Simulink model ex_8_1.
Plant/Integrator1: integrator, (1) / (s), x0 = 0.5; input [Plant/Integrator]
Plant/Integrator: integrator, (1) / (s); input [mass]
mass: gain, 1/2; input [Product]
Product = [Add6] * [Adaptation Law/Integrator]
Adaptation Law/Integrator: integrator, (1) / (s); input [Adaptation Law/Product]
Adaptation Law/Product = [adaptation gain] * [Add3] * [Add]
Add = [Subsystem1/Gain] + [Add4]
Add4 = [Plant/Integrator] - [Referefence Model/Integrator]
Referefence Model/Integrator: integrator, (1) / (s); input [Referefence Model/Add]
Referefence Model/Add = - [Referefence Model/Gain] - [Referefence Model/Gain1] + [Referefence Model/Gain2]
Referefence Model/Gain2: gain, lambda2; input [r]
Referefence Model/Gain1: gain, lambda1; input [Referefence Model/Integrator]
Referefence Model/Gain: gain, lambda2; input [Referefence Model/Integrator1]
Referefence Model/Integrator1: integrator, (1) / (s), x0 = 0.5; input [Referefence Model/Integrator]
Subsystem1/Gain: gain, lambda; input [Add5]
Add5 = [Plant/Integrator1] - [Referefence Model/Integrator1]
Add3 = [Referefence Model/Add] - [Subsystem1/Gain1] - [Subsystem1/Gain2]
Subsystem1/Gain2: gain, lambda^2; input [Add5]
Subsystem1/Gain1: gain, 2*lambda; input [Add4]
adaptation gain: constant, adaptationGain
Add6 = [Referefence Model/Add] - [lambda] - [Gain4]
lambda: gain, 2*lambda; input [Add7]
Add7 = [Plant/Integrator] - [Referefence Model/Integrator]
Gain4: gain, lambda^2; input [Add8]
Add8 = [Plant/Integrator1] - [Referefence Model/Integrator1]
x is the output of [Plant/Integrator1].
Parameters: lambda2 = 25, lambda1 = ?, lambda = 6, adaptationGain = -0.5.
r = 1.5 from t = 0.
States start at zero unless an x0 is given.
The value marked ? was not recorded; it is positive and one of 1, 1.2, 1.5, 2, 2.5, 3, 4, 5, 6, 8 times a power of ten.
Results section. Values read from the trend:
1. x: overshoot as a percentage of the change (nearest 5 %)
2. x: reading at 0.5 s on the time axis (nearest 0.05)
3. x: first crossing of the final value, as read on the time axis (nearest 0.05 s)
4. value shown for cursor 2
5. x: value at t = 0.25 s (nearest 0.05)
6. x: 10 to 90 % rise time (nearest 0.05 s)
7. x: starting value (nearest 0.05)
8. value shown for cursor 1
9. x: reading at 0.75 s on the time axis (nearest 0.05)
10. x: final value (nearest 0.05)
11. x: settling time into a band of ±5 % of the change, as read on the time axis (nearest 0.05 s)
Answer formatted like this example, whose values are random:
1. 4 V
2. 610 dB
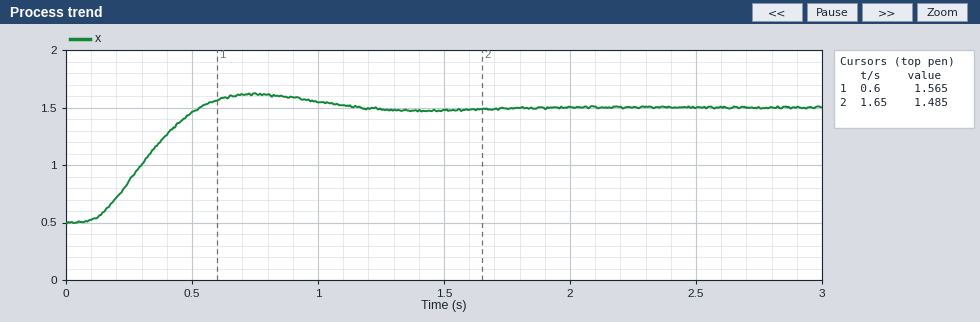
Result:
1. 10 %
2. 1.45
3. 0.55 s
4. 1.485
5. 0.85
6. 0.30 s
7. 0.50
8. 1.565
9. 1.60
10. 1.50
11. 1.00 s
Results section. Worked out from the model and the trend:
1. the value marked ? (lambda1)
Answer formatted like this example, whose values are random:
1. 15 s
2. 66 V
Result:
1. 5
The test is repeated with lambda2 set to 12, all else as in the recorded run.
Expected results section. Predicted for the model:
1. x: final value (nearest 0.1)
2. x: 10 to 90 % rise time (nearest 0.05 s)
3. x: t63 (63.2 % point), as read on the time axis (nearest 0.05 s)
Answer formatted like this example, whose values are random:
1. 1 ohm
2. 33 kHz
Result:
1. 1.5
2. 0.55 s
3. 0.55 s
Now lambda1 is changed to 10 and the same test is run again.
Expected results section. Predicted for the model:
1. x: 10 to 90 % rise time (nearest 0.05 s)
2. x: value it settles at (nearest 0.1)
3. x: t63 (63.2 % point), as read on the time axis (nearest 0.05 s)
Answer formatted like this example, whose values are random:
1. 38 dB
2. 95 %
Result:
1. 0.65 s
2. 1.5
3. 0.50 s
